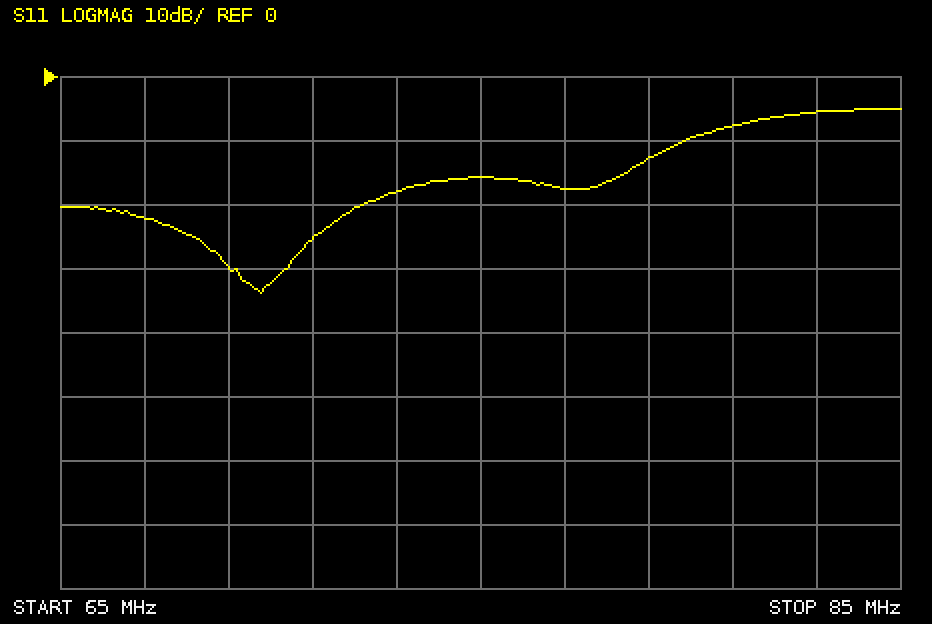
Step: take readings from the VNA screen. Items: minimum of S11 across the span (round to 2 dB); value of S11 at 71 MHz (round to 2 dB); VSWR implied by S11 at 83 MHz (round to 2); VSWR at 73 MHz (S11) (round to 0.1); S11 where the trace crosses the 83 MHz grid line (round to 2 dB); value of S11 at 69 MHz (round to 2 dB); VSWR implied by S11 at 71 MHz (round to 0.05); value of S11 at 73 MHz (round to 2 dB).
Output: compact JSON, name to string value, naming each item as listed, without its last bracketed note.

{"minimum of S11 across the span": "-34 dB", "value of S11 at 71 MHz": "-26 dB", "VSWR implied by S11 at 83 MHz": "4", "VSWR at 73 MHz (S11)": "1.3", "S11 where the trace crosses the 83 MHz grid line": "-6 dB", "value of S11 at 69 MHz": "-30 dB", "VSWR implied by S11 at 71 MHz": "1.10", "value of S11 at 73 MHz": "-18 dB"}
